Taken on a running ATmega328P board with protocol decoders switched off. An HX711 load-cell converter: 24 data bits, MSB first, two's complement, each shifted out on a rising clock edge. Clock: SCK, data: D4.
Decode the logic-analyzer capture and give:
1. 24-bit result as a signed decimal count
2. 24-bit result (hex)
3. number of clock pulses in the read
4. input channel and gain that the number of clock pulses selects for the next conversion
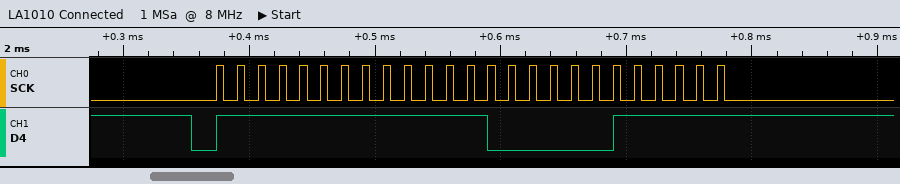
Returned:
-2017
0xFFF81F
25
channel A, gain 128
